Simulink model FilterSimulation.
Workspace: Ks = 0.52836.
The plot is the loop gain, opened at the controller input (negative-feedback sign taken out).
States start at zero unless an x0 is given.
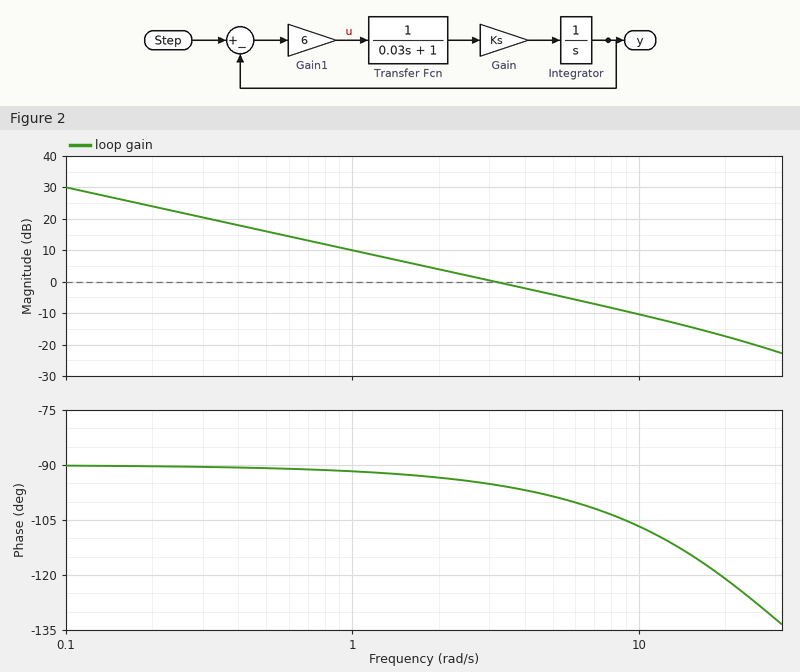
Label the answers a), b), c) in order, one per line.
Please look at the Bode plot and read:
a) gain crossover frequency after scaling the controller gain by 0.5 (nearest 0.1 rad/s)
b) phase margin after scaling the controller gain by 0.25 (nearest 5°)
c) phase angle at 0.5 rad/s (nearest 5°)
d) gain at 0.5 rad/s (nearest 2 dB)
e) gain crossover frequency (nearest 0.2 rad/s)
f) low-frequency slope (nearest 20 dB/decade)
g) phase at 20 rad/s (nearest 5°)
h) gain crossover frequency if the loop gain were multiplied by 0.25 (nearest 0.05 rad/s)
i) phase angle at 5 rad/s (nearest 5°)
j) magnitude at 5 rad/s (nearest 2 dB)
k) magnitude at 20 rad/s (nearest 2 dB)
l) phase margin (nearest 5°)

a) 1.6 rad/s
b) 90°
c) -90°
d) 16 dB
e) 3.2 rad/s
f) -20 dB/decade
g) -120°
h) 0.80 rad/s
i) -100°
j) -4 dB
k) -18 dB
l) 85°
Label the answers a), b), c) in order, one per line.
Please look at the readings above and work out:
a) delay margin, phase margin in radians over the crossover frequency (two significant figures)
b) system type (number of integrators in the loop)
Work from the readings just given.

a) 0.46 s
b) 1
